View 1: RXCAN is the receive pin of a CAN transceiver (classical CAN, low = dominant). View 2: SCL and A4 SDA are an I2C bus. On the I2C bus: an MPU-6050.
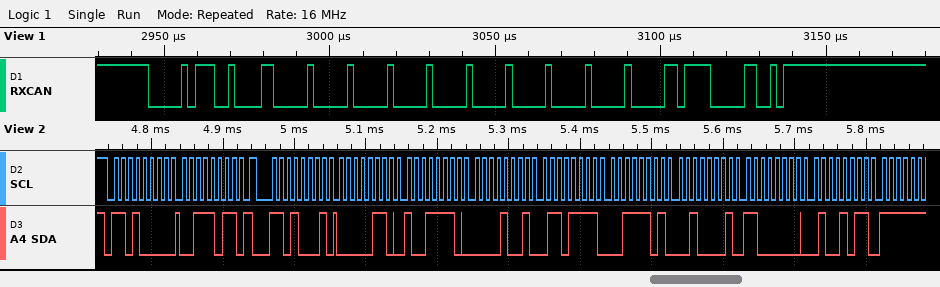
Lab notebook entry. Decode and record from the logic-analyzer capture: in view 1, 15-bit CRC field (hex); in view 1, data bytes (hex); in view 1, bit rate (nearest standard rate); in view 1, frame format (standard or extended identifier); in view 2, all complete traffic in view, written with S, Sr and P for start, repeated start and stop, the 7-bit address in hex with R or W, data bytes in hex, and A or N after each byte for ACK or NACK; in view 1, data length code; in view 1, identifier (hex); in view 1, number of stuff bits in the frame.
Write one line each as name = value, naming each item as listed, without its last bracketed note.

in view 1, 15-bit CRC field = 0x2F04
in view 1, data bytes = 00 00 00 00 00 00
in view 1, bit rate = 500 kbit/s
in view 1, frame format = standard
in view 2, all complete traffic in view, written with S, Sr and P for start, repeated start and stop, the 7-bit address in hex with R or W, data bytes in hex, and A or N after each byte for ACK or NACK = S 68W A 3B A Sr 68R A 06 A 9E A 09 A 6F A 3D A 21 A C0 A 4B A
in view 1, data length code = 6
in view 1, identifier = 0x039
in view 1, number of stuff bits in the frame = 12
